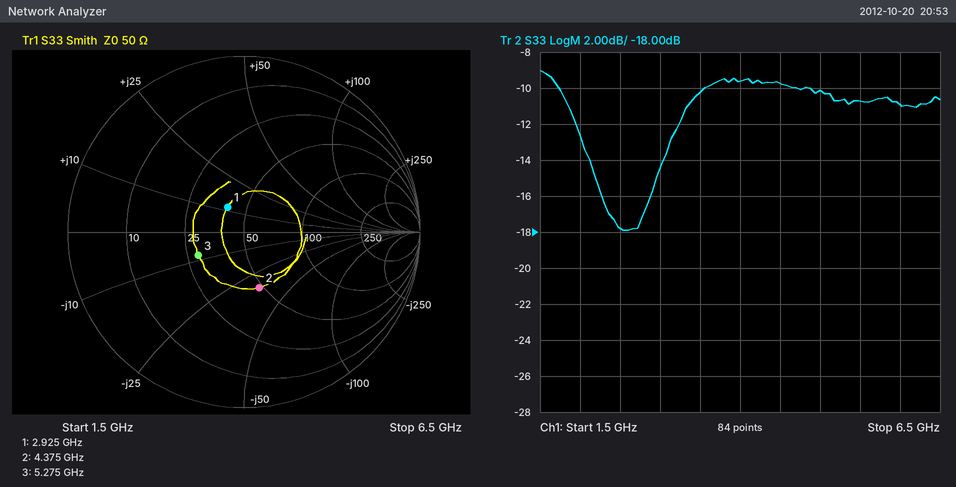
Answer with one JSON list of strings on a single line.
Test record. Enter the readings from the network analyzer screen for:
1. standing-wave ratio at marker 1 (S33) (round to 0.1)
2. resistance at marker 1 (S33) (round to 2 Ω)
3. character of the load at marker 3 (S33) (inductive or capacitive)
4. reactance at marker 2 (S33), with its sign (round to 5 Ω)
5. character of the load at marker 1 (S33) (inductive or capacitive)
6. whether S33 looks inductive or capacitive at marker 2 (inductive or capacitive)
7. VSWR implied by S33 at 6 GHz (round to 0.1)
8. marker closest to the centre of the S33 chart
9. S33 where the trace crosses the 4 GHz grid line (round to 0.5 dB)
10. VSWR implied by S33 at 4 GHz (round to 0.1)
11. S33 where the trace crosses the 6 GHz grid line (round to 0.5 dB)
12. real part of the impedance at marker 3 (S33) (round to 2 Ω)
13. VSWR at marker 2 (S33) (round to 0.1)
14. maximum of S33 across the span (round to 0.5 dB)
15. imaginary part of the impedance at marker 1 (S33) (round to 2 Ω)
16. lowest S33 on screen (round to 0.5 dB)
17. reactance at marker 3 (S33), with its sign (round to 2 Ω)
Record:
["1.4", "40 Ω", "capacitive", "-35 Ω", "inductive", "capacitive", "1.8", "marker 1", "-9.5 dB", "2.0", "-11.0 dB", "28 Ω", "2.0", "-9.0 dB", "+12 Ω", "-18.0 dB", "-8 Ω"]
